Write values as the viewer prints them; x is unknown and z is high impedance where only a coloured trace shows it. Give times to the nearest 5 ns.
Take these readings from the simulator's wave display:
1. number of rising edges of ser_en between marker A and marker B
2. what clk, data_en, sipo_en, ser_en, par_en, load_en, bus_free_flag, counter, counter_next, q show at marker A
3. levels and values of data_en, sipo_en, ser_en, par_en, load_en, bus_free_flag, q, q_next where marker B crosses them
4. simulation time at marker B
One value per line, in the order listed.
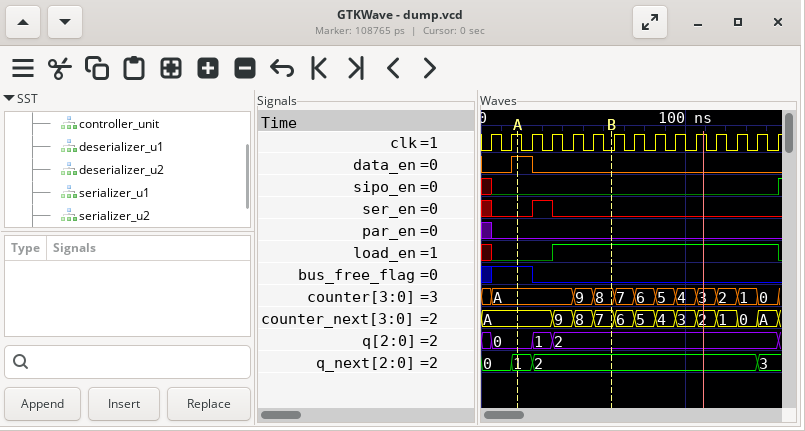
1
clk=1, data_en=1, sipo_en=0, ser_en=0, par_en=0, load_en=0, bus_free_flag=1, counter=A, counter_next=A, q=0
data_en=0, sipo_en=0, ser_en=0, par_en=0, load_en=1, bus_free_flag=0, q=2, q_next=2
65 ns
